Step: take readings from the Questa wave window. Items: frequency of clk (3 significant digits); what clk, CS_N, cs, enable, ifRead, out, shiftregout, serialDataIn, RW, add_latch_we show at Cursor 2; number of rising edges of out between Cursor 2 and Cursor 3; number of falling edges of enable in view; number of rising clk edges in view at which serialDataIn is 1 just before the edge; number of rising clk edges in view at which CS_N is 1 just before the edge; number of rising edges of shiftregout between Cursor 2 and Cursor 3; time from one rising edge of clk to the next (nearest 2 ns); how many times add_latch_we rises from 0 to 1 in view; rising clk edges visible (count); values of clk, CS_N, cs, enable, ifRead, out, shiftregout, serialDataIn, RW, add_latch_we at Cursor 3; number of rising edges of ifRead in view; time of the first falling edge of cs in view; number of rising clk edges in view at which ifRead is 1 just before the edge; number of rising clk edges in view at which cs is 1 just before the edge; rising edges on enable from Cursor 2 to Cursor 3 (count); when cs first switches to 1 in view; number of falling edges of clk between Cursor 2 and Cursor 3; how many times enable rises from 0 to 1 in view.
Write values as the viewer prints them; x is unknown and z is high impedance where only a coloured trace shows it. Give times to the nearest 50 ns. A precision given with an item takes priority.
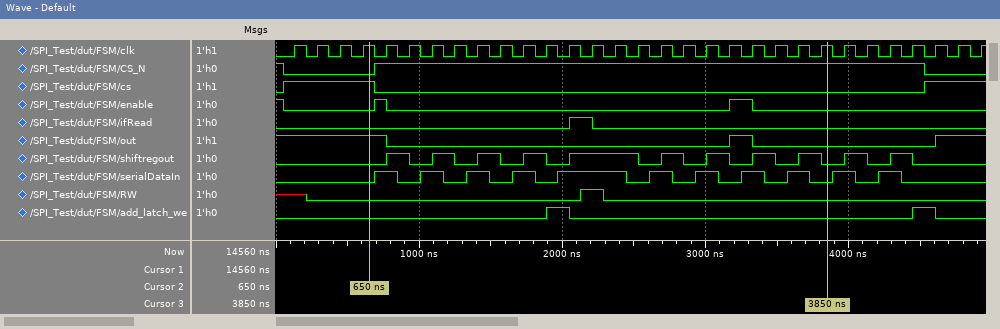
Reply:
6.25 MHz
clk=1, CS_N=0, cs=1, enable=0, ifRead=0, out=1, shiftregout=0, serialDataIn=0, RW=0, add_latch_we=0
1
3
13
24
9
160 ns
2
31
clk=1, CS_N=1, cs=0, enable=0, ifRead=0, out=0, shiftregout=0, serialDataIn=0, RW=0, add_latch_we=0
1
700 ns
1
7
2
50 ns
20
2
